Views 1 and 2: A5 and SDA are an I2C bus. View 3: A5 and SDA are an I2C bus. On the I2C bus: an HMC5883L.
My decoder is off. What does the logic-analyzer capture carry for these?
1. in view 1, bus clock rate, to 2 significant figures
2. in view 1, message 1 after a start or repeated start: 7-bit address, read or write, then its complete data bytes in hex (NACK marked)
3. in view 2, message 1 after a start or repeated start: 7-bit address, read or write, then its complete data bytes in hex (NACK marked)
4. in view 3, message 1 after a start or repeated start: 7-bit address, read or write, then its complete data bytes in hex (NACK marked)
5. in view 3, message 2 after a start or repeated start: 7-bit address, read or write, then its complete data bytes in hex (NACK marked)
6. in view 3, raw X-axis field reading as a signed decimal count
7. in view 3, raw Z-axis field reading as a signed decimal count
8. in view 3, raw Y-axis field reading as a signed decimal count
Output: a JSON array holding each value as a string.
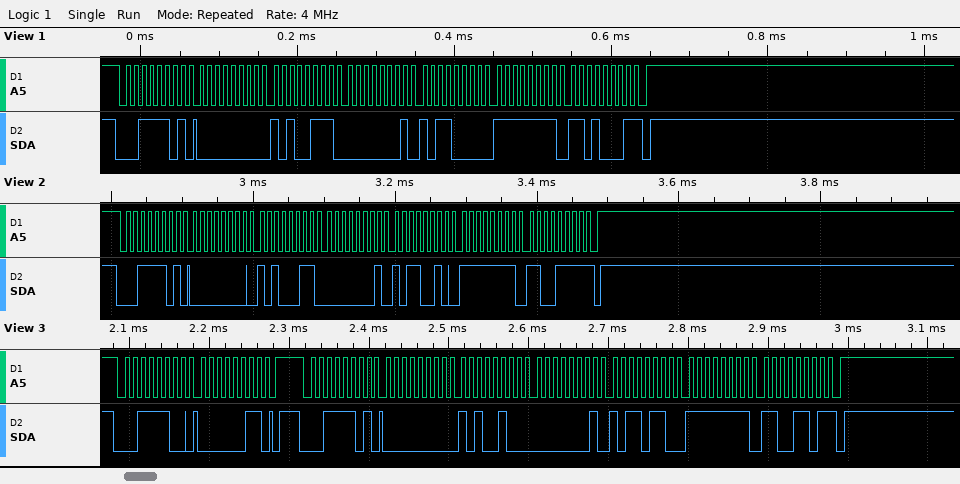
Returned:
["100 kHz", "0x1E read: 00 A7 01 B0 FF D1 NACK", "0x1E read: 00 A3 01 B2 FF CF NACK", "0x1E write: 03", "0x1E read: 00 A4 01 B6 FF CD NACK", "164", "438", "-51"]
